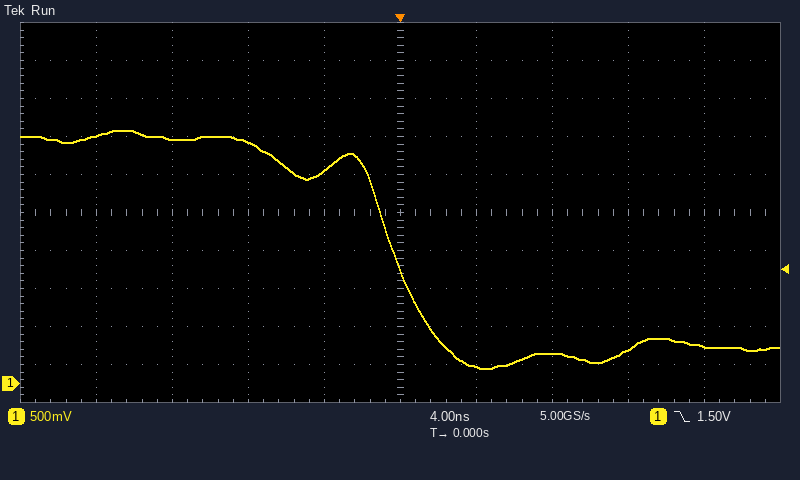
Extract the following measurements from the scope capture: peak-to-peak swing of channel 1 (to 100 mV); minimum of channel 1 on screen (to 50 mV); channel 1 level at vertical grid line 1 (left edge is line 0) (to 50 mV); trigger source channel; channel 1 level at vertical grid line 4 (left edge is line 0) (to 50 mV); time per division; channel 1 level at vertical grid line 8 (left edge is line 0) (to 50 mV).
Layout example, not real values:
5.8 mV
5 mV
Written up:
3.10 V
200 mV
3.25 V
channel 1
2.80 V
4 ns
450 mV
